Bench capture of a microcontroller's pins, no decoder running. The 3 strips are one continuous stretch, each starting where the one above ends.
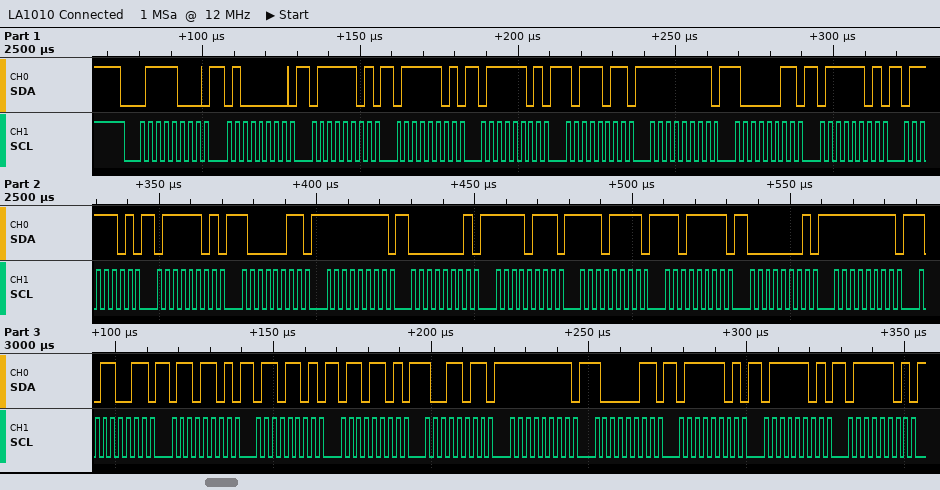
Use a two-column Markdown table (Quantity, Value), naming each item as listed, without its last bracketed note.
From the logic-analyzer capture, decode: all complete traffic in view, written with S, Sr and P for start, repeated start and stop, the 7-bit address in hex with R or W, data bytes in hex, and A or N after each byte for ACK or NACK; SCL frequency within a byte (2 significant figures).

| Quantity | Value |
|---|---|
| all complete traffic in view, written with S, Sr and P for start, repeated start and stop, the 7-bit address in hex with R or W, data bytes in hex, and A or N after each byte for ACK or NACK | S 3CW A 40 A 7D A 7D A 7D A BB A FF A 83 A 7D A 7D A 7D A 83 A FF A 01 A F7 A EF A DF A 01 A FF A B3 A 6D A 6D A 6D A 9B A FF A 83 A 7D A 7D A 7D A |
| SCL frequency within a byte | 400 kHz |
